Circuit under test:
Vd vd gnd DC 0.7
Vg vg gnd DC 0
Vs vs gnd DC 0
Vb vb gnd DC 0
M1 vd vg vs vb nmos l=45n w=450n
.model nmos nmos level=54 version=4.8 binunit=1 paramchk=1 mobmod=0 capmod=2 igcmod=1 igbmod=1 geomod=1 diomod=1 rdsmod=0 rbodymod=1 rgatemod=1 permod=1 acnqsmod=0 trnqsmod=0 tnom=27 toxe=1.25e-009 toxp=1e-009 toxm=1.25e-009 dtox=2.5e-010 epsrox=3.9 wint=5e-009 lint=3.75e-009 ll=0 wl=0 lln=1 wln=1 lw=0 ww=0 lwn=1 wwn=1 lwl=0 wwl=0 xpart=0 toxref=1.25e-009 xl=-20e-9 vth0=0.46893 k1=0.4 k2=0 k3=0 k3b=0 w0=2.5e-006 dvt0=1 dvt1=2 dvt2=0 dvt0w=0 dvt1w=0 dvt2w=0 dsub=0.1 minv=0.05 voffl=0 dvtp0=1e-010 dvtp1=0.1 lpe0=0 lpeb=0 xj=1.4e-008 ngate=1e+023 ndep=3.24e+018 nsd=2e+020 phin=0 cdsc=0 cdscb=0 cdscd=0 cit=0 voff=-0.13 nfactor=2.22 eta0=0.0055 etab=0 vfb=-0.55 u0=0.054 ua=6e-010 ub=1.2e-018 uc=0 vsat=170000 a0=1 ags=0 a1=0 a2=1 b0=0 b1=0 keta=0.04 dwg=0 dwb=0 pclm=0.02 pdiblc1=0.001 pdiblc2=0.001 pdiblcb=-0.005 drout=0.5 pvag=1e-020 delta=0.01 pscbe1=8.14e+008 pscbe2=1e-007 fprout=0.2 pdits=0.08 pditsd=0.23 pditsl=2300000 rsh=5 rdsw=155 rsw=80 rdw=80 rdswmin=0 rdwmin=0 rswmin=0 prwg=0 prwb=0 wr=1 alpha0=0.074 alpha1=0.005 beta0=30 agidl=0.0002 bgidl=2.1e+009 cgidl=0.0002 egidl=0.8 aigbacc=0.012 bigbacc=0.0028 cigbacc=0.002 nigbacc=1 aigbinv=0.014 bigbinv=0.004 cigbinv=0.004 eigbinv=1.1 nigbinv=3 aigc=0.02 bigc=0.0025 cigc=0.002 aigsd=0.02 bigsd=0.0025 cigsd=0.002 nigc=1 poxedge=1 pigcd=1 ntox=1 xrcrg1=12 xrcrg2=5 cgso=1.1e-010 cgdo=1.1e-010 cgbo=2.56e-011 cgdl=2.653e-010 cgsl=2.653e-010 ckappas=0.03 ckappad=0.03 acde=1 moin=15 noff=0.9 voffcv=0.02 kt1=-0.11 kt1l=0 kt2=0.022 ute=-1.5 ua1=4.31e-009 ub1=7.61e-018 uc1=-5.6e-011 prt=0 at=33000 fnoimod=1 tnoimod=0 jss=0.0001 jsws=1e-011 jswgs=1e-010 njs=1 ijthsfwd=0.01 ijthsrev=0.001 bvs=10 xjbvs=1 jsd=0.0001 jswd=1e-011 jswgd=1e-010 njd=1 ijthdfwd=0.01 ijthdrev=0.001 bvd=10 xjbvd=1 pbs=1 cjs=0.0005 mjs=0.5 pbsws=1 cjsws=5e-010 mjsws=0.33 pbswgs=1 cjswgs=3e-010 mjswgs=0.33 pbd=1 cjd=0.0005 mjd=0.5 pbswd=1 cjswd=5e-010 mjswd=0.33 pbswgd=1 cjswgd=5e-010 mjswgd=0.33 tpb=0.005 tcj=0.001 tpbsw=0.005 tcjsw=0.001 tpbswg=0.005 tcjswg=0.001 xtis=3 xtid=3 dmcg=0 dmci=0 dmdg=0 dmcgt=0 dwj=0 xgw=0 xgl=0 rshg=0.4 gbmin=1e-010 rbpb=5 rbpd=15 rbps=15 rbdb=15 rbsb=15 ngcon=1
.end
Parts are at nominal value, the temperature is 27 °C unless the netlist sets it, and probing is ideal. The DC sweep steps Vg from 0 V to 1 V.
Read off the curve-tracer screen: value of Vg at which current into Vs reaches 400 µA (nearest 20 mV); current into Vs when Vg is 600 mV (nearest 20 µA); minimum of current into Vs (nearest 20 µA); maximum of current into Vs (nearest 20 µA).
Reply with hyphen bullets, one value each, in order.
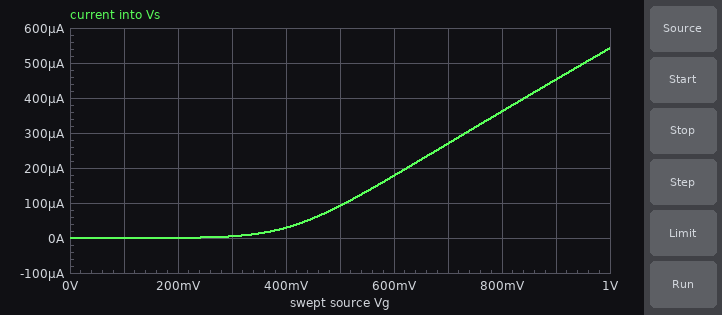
- 840 mV
- 180 µA
- 0 A
- 540 µA
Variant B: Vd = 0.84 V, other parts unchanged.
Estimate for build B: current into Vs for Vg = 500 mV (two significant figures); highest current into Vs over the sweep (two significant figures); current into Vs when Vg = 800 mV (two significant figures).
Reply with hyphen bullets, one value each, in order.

- 110 µA
- 570 µA
- 380 µA
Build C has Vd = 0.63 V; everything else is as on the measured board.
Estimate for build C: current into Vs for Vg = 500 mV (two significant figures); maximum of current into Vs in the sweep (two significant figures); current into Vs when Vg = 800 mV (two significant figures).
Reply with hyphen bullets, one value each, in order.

- 84 µA
- 530 µA
- 350 µA
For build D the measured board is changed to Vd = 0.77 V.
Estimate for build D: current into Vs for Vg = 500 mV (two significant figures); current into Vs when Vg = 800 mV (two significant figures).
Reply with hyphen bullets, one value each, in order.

- 100 µA
- 370 µA
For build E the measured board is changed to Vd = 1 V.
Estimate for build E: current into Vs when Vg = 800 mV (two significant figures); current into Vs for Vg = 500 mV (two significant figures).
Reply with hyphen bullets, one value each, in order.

- 410 µA
- 130 µA
